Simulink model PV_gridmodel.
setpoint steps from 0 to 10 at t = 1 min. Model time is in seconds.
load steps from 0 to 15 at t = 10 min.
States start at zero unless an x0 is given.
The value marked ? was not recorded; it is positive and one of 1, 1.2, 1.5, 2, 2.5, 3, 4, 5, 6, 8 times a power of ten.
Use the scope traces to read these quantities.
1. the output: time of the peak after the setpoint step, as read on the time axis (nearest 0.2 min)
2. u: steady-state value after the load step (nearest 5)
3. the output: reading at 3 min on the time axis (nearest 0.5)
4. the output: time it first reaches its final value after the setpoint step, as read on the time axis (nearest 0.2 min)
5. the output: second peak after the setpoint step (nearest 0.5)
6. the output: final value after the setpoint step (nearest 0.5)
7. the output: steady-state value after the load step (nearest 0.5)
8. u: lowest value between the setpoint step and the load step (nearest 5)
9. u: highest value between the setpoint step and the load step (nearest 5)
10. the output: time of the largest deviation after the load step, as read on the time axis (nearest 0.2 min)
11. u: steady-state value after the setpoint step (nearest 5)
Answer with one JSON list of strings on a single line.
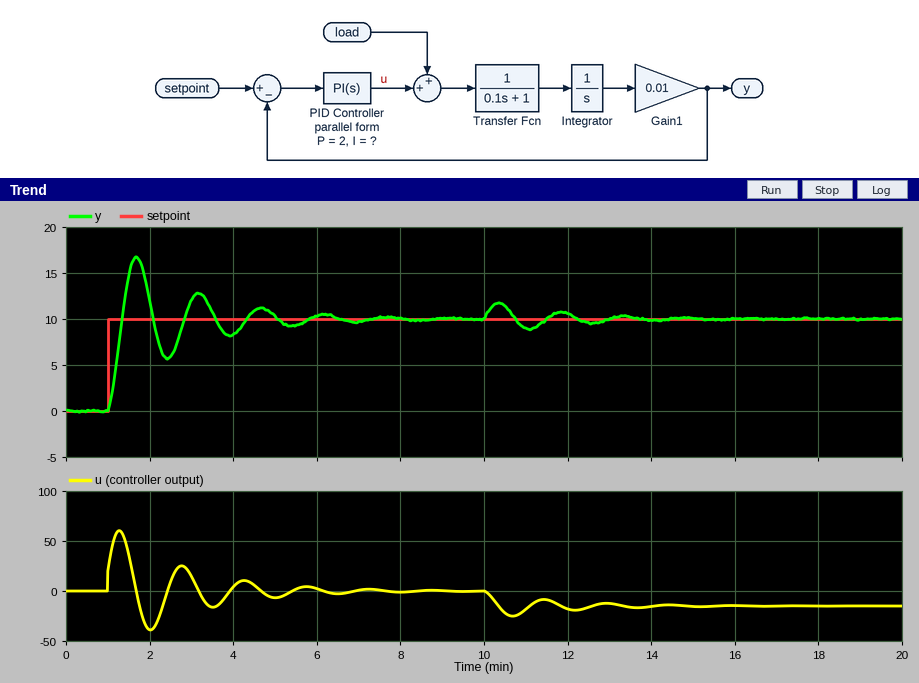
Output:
["1.6 min", "-15", "12.0", "1.4 min", "13.0", "10.0", "10.0", "-40", "60", "10.4 min", "0"]
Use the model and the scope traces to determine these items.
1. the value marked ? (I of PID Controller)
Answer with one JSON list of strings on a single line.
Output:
["0.5"]
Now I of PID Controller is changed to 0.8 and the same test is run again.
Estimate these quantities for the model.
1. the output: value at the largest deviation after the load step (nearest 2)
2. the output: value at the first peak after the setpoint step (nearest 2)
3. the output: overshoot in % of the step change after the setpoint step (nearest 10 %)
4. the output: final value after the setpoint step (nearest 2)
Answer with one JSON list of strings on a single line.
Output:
["12", "18", "70 %", "10"]
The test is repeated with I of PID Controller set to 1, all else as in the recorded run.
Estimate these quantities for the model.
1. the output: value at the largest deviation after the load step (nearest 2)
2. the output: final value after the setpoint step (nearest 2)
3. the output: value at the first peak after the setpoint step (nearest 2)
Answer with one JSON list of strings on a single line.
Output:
["12", "10", "18"]
